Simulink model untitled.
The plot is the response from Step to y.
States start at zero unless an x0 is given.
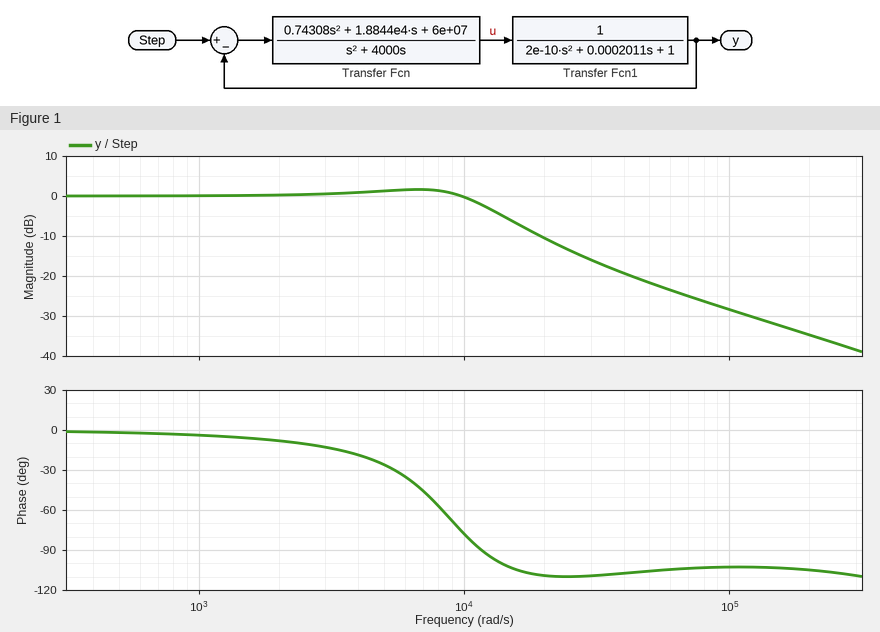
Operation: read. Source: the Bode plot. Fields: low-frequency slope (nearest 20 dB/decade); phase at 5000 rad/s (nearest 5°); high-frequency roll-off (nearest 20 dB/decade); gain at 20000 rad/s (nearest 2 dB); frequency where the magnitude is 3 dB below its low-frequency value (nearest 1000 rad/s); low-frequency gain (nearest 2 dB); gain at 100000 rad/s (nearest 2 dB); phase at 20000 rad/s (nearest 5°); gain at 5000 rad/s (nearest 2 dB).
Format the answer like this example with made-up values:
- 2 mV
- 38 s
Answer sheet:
- 0 dB/decade
- -25°
- -20 dB/decade
- -10 dB
- 12000 rad/s
- 0 dB
- -28 dB
- -110°
- 2 dB
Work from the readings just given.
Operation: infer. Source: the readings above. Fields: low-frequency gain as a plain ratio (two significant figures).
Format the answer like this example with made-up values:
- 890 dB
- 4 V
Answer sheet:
- 1.0
